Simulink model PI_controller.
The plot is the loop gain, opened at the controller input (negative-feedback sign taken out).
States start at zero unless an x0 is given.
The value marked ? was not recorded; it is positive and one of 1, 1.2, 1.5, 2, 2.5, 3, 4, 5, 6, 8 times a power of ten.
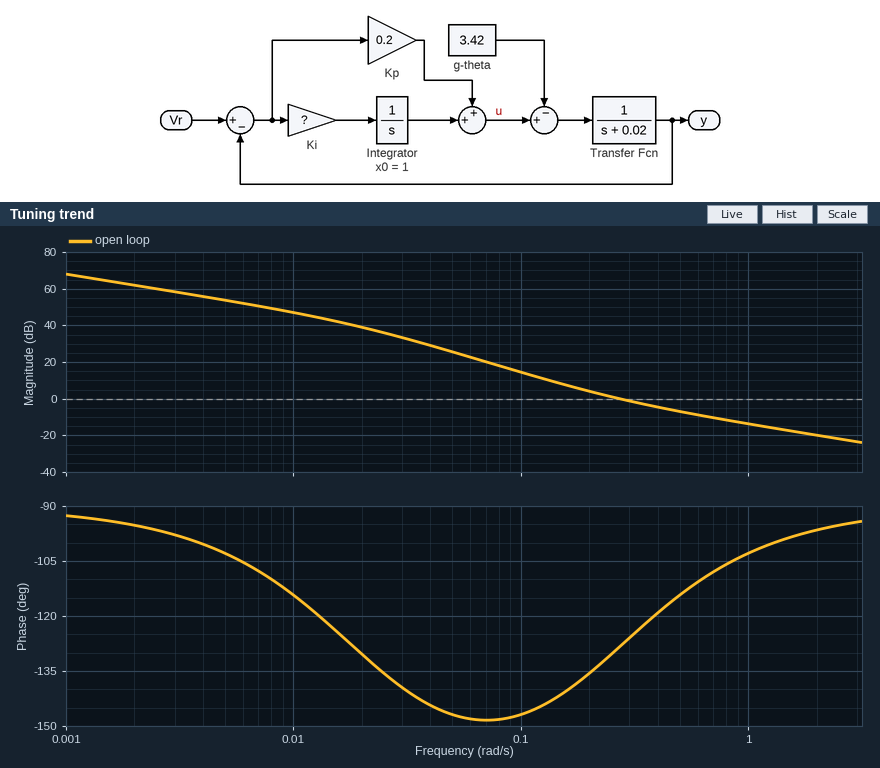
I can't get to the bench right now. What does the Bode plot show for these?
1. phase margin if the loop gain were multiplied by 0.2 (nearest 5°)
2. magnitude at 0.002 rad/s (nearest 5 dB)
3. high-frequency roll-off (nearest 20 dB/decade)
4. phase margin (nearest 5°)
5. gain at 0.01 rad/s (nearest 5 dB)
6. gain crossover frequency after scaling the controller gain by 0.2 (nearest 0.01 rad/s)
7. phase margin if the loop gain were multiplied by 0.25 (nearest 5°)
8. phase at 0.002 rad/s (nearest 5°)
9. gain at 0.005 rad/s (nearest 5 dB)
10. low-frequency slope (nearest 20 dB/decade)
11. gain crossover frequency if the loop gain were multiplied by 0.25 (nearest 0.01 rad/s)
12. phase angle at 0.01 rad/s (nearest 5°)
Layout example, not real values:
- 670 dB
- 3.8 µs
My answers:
- 35°
- 60 dB
- -20 dB/decade
- 50°
- 45 dB
- 0.10 rad/s
- 35°
- -95°
- 55 dB
- -20 dB/decade
- 0.12 rad/s
- -115°
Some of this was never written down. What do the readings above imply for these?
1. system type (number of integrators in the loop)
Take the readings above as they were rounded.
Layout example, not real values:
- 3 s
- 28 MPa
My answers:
- 1
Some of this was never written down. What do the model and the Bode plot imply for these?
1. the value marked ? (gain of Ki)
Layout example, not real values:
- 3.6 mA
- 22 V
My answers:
- 0.05
